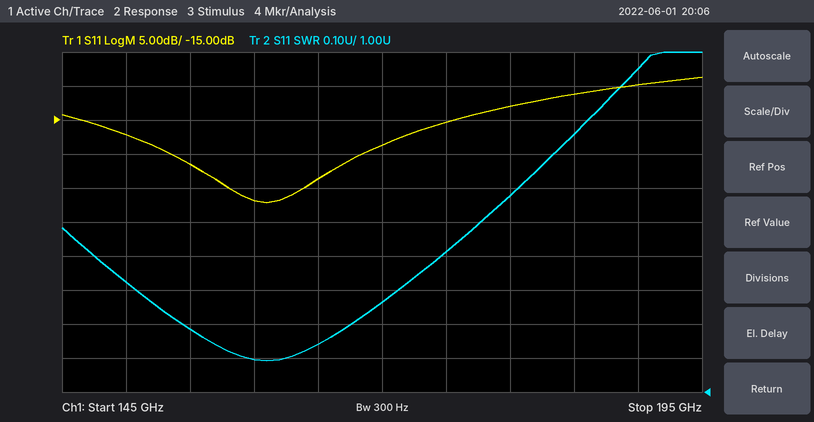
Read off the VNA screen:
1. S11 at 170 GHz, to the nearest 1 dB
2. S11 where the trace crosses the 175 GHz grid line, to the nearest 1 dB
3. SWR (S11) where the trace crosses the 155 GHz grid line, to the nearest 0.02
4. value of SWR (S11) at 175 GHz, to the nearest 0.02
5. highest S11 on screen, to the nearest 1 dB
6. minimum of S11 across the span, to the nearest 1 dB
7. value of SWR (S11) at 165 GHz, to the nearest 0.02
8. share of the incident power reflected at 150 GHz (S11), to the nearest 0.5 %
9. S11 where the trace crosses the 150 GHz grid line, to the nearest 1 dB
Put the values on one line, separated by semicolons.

-19 dB; -15 dB; 1.18; 1.42; -9 dB; -27 dB; 1.14; 2.0 %; -17 dB
